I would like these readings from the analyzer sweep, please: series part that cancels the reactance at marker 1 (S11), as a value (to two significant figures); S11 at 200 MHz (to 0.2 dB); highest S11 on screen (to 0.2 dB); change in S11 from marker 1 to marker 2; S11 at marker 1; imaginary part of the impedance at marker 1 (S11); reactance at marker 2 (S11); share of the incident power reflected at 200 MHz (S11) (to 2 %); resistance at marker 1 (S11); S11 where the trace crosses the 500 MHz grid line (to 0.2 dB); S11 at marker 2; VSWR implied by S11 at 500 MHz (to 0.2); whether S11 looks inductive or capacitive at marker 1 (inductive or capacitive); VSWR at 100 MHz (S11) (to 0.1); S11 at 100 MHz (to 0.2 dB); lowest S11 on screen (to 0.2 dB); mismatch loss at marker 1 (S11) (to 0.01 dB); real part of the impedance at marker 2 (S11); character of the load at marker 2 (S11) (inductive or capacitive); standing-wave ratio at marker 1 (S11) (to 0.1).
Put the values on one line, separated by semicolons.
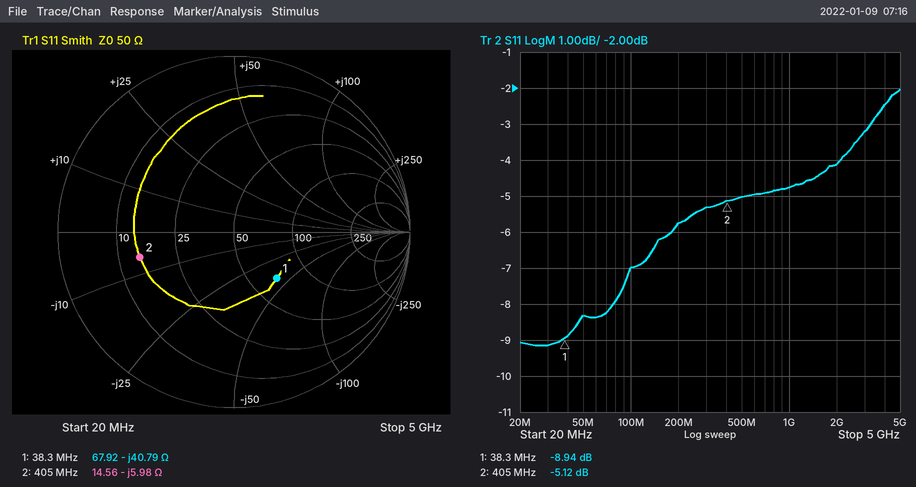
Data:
170 nH; -5.8 dB; -2.0 dB; 3.82 dB; -8.94 dB; -40.79 Ω; -5.98 Ω; 26 %; 67.92 Ω; -5.0 dB; -5.12 dB; 3.6; capacitive; 2.6; -7.0 dB; -9.2 dB; 0.59 dB; 14.56 Ω; capacitive; 2.1
